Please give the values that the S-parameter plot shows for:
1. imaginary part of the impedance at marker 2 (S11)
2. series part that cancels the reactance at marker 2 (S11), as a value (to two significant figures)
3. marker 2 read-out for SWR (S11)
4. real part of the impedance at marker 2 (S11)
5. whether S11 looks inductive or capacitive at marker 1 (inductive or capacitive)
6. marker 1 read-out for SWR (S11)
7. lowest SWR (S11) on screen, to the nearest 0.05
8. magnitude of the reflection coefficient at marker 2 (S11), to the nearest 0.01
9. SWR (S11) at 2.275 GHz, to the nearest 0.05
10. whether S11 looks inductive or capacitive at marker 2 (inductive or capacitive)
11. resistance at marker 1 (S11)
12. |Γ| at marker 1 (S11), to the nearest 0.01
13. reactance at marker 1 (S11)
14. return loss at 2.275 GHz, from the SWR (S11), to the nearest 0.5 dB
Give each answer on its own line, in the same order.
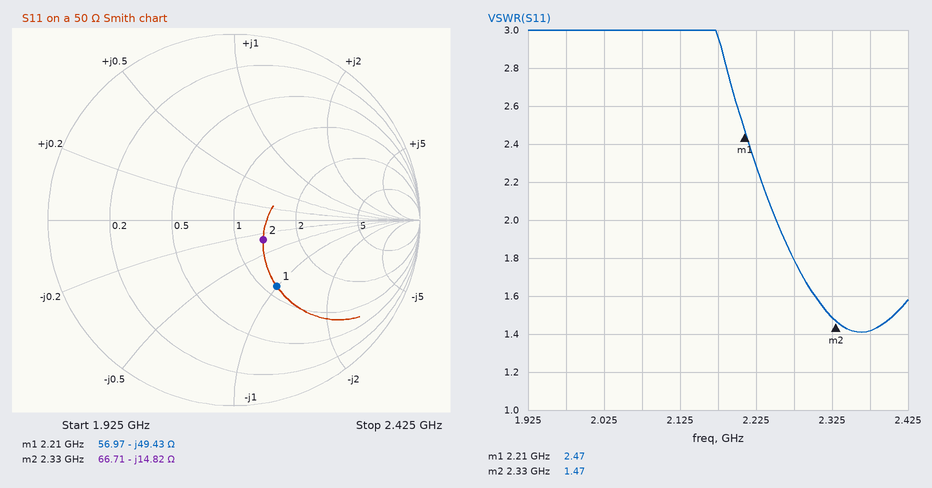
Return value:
-14.82 Ω
1.0 nH
1.47
66.71 Ω
capacitive
2.47
1.40
0.19
1.80
capacitive
56.97 Ω
0.42
-49.43 Ω
11.0 dB
